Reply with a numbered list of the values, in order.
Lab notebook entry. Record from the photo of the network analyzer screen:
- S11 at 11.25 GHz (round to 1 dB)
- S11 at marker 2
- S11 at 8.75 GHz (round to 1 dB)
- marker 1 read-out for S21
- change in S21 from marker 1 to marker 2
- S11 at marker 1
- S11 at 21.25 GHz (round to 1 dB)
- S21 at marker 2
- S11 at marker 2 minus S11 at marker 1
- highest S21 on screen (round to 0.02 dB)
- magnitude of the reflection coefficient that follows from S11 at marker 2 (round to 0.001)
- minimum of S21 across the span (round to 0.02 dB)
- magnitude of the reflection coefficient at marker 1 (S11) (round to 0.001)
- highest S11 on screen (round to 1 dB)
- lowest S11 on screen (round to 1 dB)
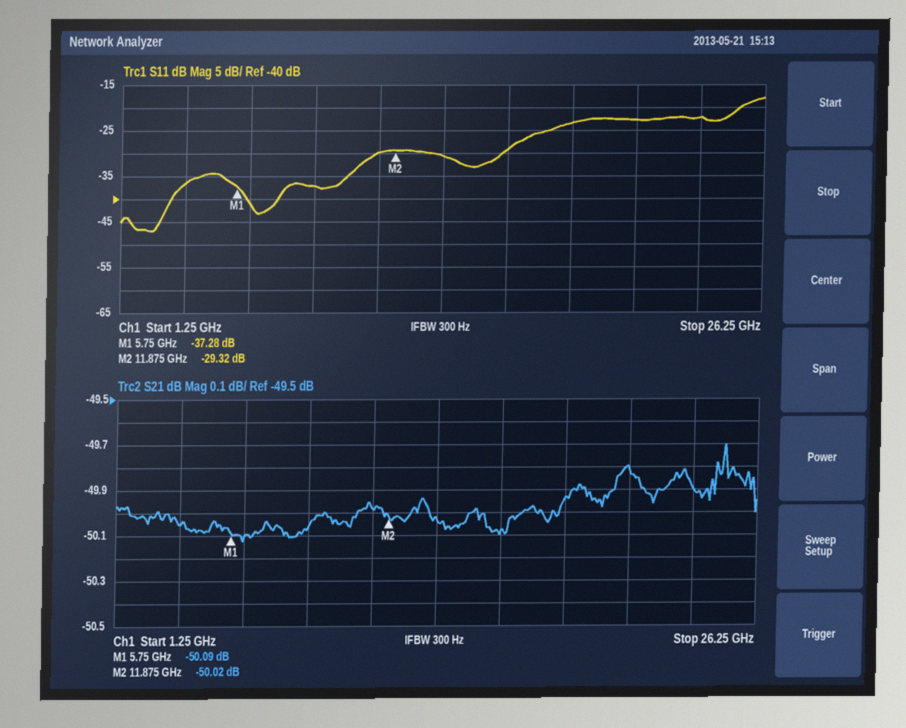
1. -30 dB
2. -29.32 dB
3. -37 dB
4. -50.09 dB
5. 0.07 dB
6. -37.28 dB
7. -23 dB
8. -50.02 dB
9. 7.96 dB
10. -49.70 dB
11. 0.034
12. -50.12 dB
13. 0.014
14. -18 dB
15. -47 dB
